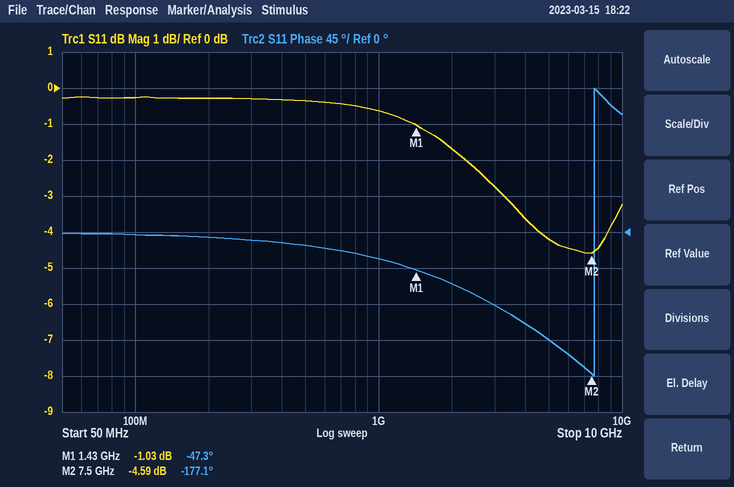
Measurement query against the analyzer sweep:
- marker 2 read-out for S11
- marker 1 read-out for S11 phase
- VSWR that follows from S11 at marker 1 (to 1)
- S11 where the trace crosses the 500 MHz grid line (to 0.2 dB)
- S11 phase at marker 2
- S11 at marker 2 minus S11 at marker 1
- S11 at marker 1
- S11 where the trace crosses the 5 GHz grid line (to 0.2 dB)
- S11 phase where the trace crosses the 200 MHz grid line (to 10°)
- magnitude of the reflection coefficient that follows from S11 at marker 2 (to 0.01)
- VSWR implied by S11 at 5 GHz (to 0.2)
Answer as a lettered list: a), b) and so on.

a) -4.59 dB
b) -47.3°
c) 17
d) -0.4 dB
e) -177.1°
f) -3.56 dB
g) -1.03 dB
h) -4.2 dB
i) -10°
j) 0.59
k) 4.2
